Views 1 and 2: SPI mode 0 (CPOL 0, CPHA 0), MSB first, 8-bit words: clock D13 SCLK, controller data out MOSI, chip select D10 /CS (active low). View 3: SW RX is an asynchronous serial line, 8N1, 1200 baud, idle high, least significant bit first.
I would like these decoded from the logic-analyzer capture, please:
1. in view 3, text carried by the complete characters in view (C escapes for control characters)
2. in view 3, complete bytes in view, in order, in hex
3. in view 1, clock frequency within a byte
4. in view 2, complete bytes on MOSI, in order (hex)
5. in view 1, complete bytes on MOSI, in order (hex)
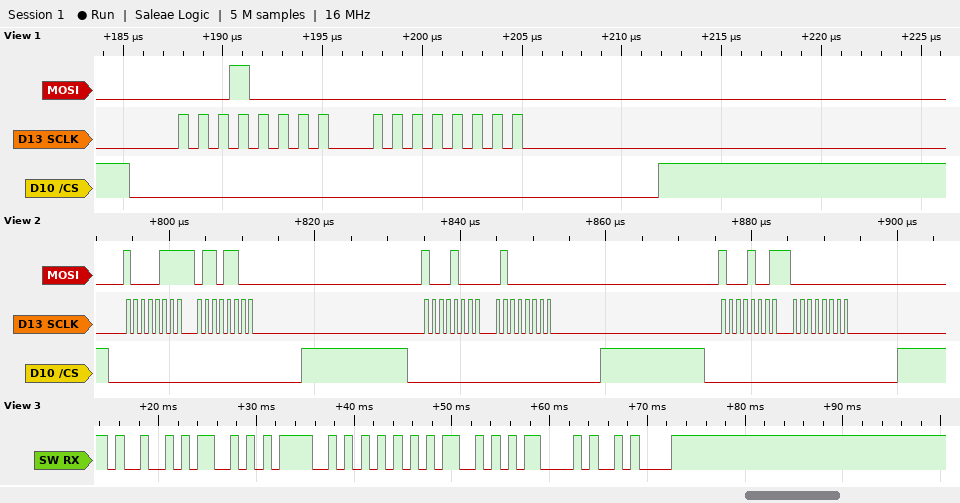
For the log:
"ISOUSC\n"
49 53 4F 55 53 43 0A
1 MHz
87 6C 88 40 89 00
10 00
